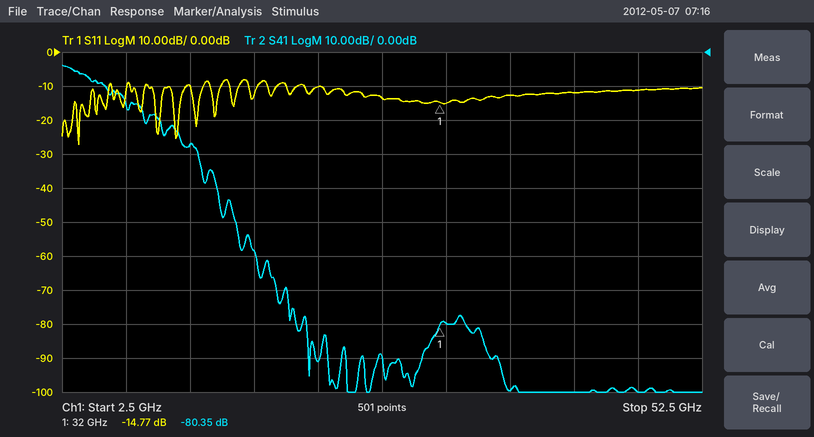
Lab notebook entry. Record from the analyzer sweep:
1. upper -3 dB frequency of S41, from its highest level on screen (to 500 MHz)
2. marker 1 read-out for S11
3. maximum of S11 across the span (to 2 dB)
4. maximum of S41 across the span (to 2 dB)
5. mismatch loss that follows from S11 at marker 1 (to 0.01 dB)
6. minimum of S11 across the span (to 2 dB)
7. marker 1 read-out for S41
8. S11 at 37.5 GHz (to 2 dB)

4.5 GHz
-14.77 dB
-8 dB
-4 dB
0.15 dB
-28 dB
-80.35 dB
-12 dB
